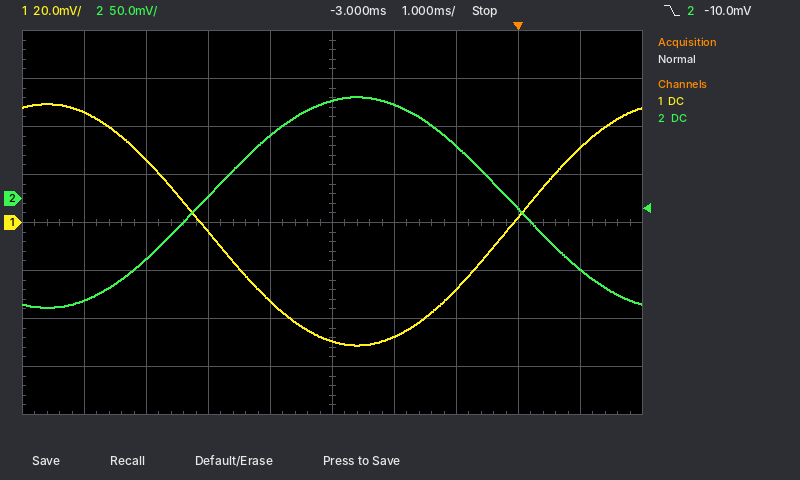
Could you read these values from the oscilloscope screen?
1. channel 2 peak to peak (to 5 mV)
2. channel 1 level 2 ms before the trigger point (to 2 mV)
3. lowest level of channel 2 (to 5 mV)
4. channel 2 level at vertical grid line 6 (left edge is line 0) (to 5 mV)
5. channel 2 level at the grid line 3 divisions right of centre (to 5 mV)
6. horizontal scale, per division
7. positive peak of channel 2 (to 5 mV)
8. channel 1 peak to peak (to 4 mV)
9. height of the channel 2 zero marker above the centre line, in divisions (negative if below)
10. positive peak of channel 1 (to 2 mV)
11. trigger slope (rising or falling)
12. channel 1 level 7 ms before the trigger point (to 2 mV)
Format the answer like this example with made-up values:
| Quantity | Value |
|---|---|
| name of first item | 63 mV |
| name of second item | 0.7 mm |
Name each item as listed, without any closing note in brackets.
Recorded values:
| Quantity | Value |
|---|---|
| channel 2 peak to peak | 220 mV |
| channel 1 level 2 ms before the trigger point | -48 mV |
| lowest level of channel 2 | -115 mV |
| channel 2 level at vertical grid line 6 (left edge is line 0) | 100 mV |
| channel 2 level at the grid line 3 divisions right of centre | -10 mV |
| horizontal scale, per division | 1 ms |
| positive peak of channel 2 | 105 mV |
| channel 1 peak to peak | 100 mV |
| height of the channel 2 zero marker above the centre line, in divisions | +0.5 div |
| positive peak of channel 1 | 50 mV |
| trigger slope | falling |
| channel 1 level 7 ms before the trigger point | 46 mV |
